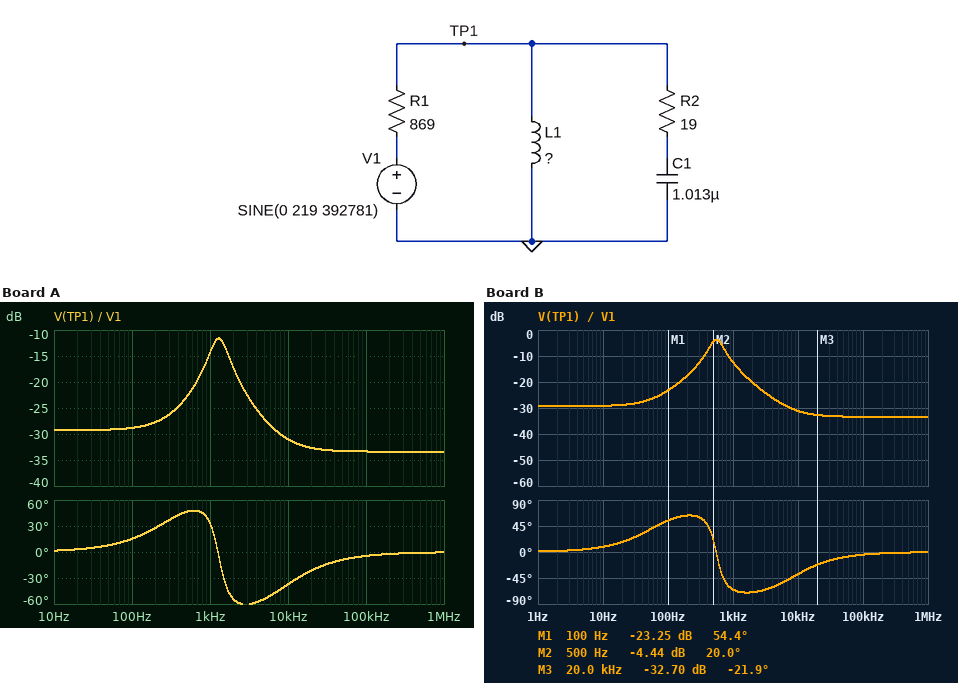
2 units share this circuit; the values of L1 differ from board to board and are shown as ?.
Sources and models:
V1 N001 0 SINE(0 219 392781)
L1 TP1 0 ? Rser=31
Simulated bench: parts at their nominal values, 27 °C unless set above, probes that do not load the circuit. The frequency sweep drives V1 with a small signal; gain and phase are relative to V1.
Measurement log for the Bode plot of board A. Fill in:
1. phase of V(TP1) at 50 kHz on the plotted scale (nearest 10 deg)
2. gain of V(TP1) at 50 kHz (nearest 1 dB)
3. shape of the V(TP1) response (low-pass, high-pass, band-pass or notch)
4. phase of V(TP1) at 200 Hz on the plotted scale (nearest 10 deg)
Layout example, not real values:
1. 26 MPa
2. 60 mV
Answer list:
1. -10 deg
2. -33 dB
3. band-pass
4. 30 deg
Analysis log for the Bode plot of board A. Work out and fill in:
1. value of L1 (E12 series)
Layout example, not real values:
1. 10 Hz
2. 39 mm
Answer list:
1. 15 mH
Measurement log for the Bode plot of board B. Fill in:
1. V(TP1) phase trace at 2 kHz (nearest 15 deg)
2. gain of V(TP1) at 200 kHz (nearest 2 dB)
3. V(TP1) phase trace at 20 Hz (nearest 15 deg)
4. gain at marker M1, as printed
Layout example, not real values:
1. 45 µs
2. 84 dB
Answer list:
1. -75 deg
2. -34 dB
3. 15 deg
4. -23.25 dB
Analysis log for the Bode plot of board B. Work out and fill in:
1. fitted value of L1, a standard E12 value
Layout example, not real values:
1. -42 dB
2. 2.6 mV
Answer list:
1. 82 mH
